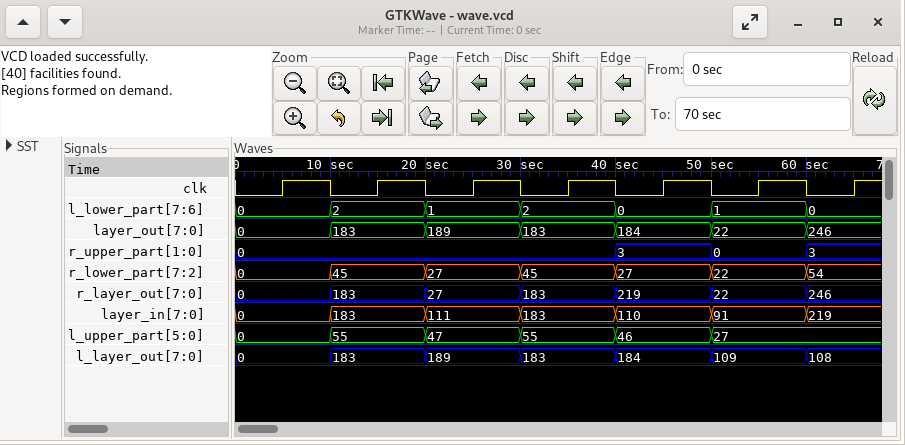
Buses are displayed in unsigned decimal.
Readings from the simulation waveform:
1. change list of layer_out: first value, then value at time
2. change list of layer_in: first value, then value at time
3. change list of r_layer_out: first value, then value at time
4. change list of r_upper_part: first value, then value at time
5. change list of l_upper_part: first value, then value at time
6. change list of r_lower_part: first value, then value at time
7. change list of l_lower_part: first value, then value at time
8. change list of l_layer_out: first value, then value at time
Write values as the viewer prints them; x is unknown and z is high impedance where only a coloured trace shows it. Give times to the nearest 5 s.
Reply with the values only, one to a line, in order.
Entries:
0, 183 at 10 s, 189 at 20 s, 183 at 30 s, 184 at 40 s, 22 at 50 s, 246 at 60 s
0, 183 at 10 s, 111 at 20 s, 183 at 30 s, 110 at 40 s, 91 at 50 s, 219 at 60 s
0, 183 at 10 s, 27 at 20 s, 183 at 30 s, 219 at 40 s, 22 at 50 s, 246 at 60 s
0, 3 at 40 s, 0 at 50 s, 3 at 60 s
0, 55 at 10 s, 47 at 20 s, 55 at 30 s, 46 at 40 s, 27 at 50 s
0, 45 at 10 s, 27 at 20 s, 45 at 30 s, 27 at 40 s, 22 at 50 s, 54 at 60 s
0, 2 at 10 s, 1 at 20 s, 2 at 30 s, 0 at 40 s, 1 at 50 s, 0 at 60 s
0, 183 at 10 s, 189 at 20 s, 183 at 30 s, 184 at 40 s, 109 at 50 s, 108 at 60 s
